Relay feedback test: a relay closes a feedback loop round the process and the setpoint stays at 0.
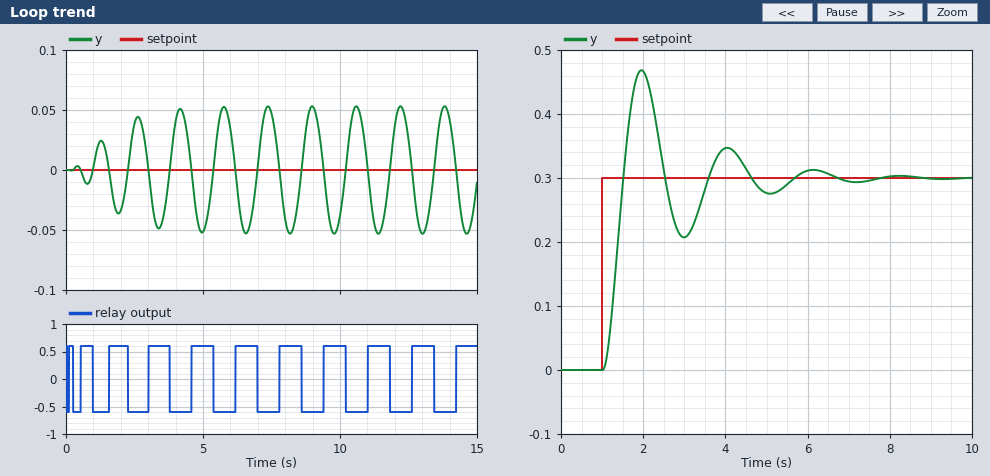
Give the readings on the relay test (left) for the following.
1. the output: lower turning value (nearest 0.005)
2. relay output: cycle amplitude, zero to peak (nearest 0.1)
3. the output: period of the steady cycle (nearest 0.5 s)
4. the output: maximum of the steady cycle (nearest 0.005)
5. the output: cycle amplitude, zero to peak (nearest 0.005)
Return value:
-0.055
0.6
1.5 s
0.055
0.055
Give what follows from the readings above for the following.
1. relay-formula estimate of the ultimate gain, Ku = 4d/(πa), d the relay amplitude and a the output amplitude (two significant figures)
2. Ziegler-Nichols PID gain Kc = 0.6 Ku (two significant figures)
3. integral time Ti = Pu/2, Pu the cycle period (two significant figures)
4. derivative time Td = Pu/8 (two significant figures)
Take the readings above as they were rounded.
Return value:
14
8.4
0.75 s
0.19 s
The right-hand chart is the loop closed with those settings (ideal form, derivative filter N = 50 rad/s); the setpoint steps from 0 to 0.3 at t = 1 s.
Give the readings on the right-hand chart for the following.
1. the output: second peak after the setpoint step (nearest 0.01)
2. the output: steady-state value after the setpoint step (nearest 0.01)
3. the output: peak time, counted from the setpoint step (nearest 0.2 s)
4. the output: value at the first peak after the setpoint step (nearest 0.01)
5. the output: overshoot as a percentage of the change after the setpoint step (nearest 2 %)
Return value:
0.35
0.30
1.0 s
0.47
56 %
